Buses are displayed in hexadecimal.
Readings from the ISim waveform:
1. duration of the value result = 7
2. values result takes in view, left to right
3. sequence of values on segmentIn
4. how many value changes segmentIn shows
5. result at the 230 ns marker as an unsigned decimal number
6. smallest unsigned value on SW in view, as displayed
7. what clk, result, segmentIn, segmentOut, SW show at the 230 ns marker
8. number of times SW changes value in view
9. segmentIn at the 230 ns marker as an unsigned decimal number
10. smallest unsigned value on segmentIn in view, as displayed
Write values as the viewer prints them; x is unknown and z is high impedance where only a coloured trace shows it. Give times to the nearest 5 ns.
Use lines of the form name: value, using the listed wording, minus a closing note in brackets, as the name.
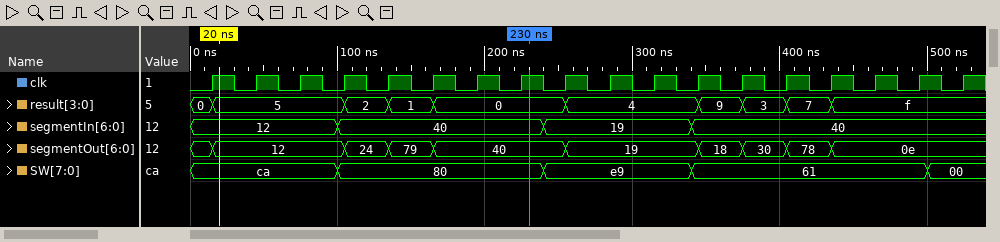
duration of the value result = 7: 30 ns
values result takes in view, left to right: 0, 5, 2, 1, 0, 4, 9, 3, 7, f
sequence of values on segmentIn: 12, 40, 19, 40
how many value changes segmentIn shows: 3
result at the 230 ns marker as an unsigned decimal number: 0
smallest unsigned value on SW in view, as displayed: 00
what clk, result, segmentIn, segmentOut, SW show at the 230 ns marker: clk=1, result=0, segmentIn=40, segmentOut=40, SW=80
number of times SW changes value in view: 4
segmentIn at the 230 ns marker as an unsigned decimal number: 64
smallest unsigned value on segmentIn in view, as displayed: 12
